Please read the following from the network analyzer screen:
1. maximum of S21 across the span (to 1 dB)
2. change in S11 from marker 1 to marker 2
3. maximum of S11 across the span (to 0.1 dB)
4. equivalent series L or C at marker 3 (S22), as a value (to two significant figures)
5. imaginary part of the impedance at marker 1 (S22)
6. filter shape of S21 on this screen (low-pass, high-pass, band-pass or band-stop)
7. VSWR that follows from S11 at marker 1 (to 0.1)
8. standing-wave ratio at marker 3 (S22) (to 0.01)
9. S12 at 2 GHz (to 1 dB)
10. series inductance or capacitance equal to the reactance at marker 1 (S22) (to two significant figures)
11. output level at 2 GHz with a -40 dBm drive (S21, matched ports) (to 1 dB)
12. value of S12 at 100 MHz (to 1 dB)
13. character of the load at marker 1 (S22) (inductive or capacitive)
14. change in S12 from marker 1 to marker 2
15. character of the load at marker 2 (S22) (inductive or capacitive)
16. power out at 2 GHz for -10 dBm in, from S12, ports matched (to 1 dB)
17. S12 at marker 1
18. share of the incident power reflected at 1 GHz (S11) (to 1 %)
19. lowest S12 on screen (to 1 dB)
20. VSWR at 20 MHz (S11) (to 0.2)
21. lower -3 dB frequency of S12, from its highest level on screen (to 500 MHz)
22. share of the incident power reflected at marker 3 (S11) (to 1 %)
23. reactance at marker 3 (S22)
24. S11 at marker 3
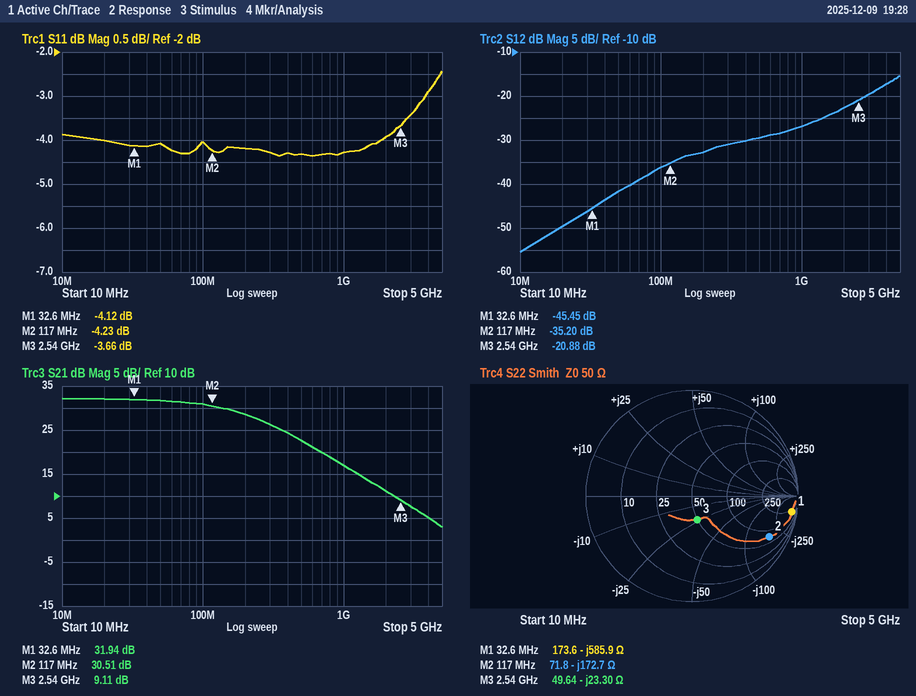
32 dB
-0.11 dB
-2.4 dB
2.7 pF
-585.9 Ω
low-pass
4.3
1.59
-23 dB
8.3 pF
-29 dBm
-36 dB
capacitive
10.25 dB
capacitive
-33 dBm
-45.45 dB
37 %
-55 dB
4.4
3.5 GHz
43 %
-23.30 Ω
-3.66 dB
